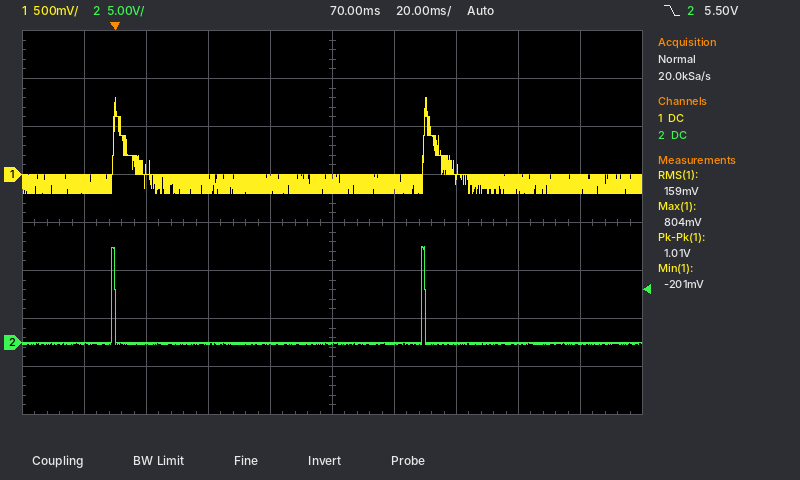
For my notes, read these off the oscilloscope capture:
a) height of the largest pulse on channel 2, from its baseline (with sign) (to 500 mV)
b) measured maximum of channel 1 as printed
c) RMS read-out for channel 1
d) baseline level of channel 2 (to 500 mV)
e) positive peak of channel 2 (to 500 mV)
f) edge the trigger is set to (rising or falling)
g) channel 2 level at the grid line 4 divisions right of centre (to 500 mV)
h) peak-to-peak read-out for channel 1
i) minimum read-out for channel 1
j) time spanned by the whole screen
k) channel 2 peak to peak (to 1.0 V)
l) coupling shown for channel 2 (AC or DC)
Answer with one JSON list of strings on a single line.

["+10.0 V", "804 mV", "159 mV", "0.0 V", "10.0 V", "falling", "0.0 V", "1.01 V", "-201 mV", "200 ms", "10.0 V", "DC"]
